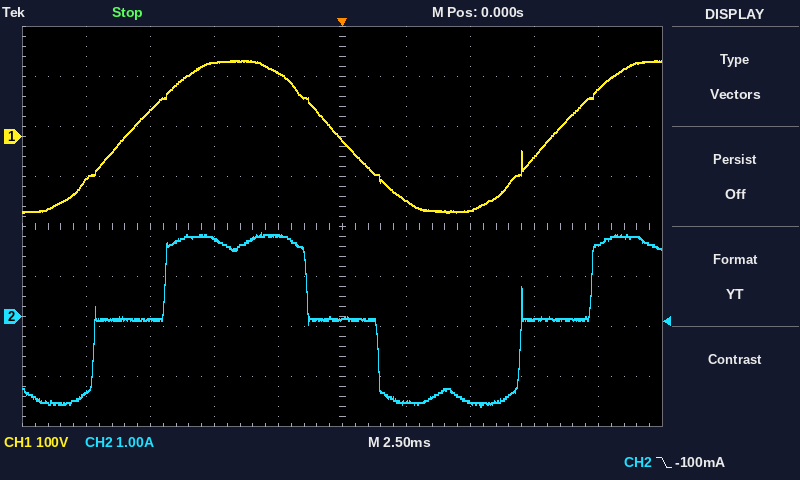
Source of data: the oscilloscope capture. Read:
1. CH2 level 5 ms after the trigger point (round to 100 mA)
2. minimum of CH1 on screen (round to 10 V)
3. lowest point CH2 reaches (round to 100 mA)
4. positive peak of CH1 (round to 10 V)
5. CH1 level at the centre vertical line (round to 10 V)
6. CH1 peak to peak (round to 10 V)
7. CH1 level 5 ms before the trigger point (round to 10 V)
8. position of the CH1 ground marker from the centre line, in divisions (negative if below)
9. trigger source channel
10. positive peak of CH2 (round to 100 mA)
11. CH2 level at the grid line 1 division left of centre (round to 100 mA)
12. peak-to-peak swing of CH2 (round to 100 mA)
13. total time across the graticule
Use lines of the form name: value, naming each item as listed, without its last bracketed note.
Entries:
CH2 level 5 ms after the trigger point: -1.7 A
minimum of CH1 on screen: -150 V
lowest point CH2 reaches: -1.8 A
positive peak of CH1: 150 V
CH1 level at the centre vertical line: -10 V
CH1 peak to peak: 300 V
CH1 level 5 ms before the trigger point: 150 V
position of the CH1 ground marker from the centre line, in divisions: +1.8 div
trigger source channel: CH2
positive peak of CH2: 1.7 A
CH2 level at the grid line 1 division left of centre: 1.6 A
peak-to-peak swing of CH2: 3.5 A
total time across the graticule: 25 ms
